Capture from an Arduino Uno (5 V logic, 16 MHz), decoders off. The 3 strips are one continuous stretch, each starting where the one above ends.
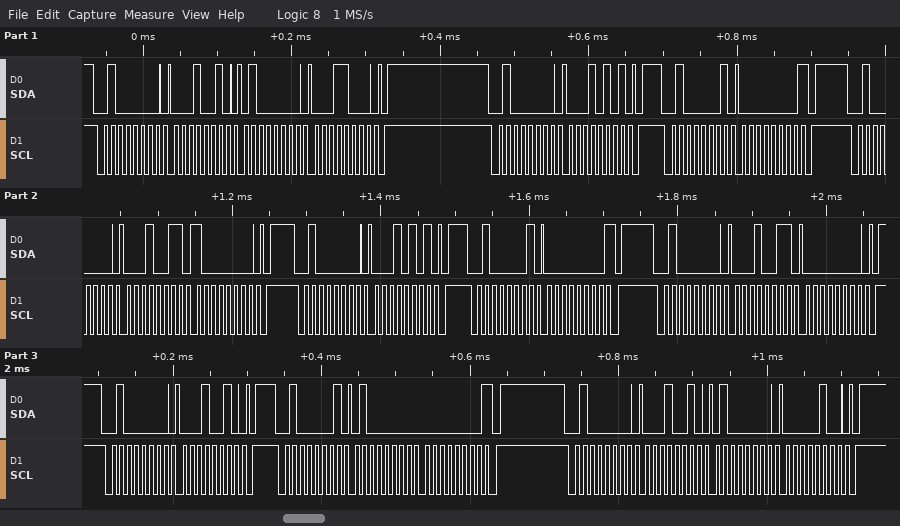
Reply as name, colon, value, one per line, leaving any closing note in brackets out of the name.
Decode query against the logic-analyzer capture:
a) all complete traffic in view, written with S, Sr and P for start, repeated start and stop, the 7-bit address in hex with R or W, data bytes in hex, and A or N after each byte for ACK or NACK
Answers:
all complete traffic in view, written with S, Sr and P for start, repeated start and stop, the 7-bit address in hex with R or W, data bytes in hex, and A or N after each byte for ACK or NACK: S 20W A 12 A 40 A 18 A P S 20W A 15 A P S 20R A 00 N P S 20W A 13 A 80 A P S 20W A 15 A P S 20R A 00 N P S 20W A 13 A 00 A P S 20W A 12 A P S 20R A 40 A 00 N P S 20W A 12 A 40 A 04 A P
